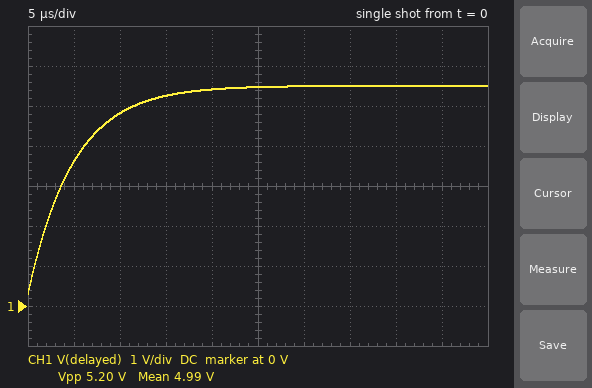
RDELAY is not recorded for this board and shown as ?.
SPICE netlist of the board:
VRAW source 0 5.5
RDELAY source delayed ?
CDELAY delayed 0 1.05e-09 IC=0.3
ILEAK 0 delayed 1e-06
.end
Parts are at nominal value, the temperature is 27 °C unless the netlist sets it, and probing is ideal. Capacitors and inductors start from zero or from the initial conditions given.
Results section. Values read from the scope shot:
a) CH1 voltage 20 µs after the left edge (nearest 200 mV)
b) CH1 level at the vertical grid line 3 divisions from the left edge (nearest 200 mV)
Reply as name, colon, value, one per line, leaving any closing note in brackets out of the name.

CH1 voltage 20 µs after the left edge: 5.4 V
CH1 level at the vertical grid line 3 divisions from the left edge: 5.2 V
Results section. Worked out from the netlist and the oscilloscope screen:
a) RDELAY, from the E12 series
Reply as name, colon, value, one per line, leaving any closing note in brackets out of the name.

RDELAY, from the E12 series: 4.7 kΩ
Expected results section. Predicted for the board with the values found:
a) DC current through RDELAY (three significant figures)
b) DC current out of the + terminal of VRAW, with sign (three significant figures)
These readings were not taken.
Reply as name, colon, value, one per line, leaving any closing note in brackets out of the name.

DC current through RDELAY: 1.00 µA
DC current out of the + terminal of VRAW, with sign: -1.00 µA
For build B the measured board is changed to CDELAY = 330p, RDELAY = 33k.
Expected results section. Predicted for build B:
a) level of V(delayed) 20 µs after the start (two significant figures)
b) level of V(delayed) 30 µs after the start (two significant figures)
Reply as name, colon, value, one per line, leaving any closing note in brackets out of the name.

level of V(delayed) 20 µs after the start: 4.7 V
level of V(delayed) 30 µs after the start: 5.2 V
